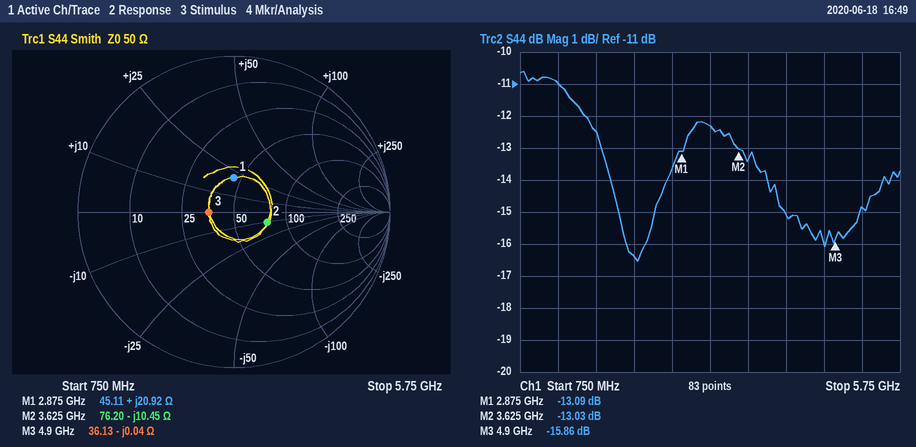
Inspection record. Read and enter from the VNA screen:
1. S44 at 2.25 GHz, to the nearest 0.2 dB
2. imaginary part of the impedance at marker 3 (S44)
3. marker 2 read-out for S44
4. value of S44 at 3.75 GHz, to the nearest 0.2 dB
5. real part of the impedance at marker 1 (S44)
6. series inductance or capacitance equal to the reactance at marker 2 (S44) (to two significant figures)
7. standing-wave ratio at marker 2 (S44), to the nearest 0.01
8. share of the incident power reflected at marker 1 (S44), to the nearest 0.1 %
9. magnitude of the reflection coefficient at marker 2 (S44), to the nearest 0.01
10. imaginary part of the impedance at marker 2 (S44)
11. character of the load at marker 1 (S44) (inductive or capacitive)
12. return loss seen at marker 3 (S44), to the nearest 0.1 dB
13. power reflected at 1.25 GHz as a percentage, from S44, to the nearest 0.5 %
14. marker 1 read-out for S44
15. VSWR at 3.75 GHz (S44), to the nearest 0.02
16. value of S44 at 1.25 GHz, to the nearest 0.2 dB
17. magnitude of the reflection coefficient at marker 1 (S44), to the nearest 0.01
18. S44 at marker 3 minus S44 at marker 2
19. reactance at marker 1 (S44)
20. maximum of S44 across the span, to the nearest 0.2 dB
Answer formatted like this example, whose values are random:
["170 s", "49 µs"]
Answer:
["-16.4 dB", "-0.04 Ω", "-13.03 dB", "-13.4 dB", "45.11 Ω", "4.2 pF", "1.57", "4.9 %", "0.22", "-10.45 Ω", "inductive", "15.9 dB", "8.0 %", "-13.09 dB", "1.54", "-11.0 dB", "0.22", "-2.83 dB", "+20.92 Ω", "-10.6 dB"]
